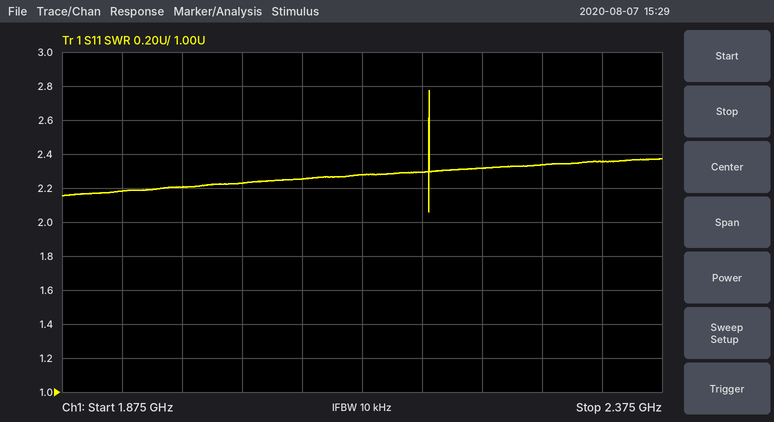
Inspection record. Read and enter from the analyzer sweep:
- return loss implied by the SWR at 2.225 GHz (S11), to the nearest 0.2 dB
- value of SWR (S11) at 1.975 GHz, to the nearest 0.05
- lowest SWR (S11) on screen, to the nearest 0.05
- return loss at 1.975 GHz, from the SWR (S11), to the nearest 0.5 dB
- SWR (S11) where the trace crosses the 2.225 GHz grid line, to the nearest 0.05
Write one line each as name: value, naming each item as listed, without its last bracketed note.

return loss implied by the SWR at 2.225 GHz (S11), to the nearest 0.2 dB: 8.0 dB
value of SWR (S11) at 1.975 GHz, to the nearest 0.05: 2.20
lowest SWR (S11) on screen, to the nearest 0.05: 2.05
return loss at 1.975 GHz, from the SWR (S11), to the nearest 0.5 dB: 8.5 dB
SWR (S11) where the trace crosses the 2.225 GHz grid line, to the nearest 0.05: 2.30
